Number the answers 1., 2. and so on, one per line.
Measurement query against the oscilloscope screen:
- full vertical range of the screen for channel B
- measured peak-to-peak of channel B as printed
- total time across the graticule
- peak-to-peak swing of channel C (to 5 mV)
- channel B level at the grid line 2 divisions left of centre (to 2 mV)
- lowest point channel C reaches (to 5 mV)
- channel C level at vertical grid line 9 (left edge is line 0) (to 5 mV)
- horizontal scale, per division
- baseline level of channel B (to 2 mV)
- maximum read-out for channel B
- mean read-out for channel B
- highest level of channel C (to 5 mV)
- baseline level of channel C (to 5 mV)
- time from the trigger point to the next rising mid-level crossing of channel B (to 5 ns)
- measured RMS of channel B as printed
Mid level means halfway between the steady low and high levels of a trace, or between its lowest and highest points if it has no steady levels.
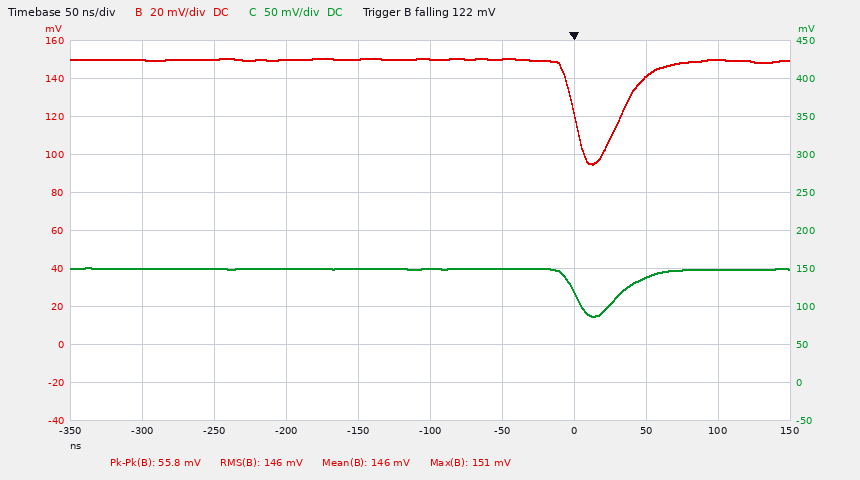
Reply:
1. 200 mV
2. 55.8 mV
3. 500 ns
4. 65 mV
5. 150 mV
6. 85 mV
7. 150 mV
8. 50 ns
9. 150 mV
10. 151 mV
11. 146 mV
12. 150 mV
13. 150 mV
14. 35 ns
15. 146 mV
